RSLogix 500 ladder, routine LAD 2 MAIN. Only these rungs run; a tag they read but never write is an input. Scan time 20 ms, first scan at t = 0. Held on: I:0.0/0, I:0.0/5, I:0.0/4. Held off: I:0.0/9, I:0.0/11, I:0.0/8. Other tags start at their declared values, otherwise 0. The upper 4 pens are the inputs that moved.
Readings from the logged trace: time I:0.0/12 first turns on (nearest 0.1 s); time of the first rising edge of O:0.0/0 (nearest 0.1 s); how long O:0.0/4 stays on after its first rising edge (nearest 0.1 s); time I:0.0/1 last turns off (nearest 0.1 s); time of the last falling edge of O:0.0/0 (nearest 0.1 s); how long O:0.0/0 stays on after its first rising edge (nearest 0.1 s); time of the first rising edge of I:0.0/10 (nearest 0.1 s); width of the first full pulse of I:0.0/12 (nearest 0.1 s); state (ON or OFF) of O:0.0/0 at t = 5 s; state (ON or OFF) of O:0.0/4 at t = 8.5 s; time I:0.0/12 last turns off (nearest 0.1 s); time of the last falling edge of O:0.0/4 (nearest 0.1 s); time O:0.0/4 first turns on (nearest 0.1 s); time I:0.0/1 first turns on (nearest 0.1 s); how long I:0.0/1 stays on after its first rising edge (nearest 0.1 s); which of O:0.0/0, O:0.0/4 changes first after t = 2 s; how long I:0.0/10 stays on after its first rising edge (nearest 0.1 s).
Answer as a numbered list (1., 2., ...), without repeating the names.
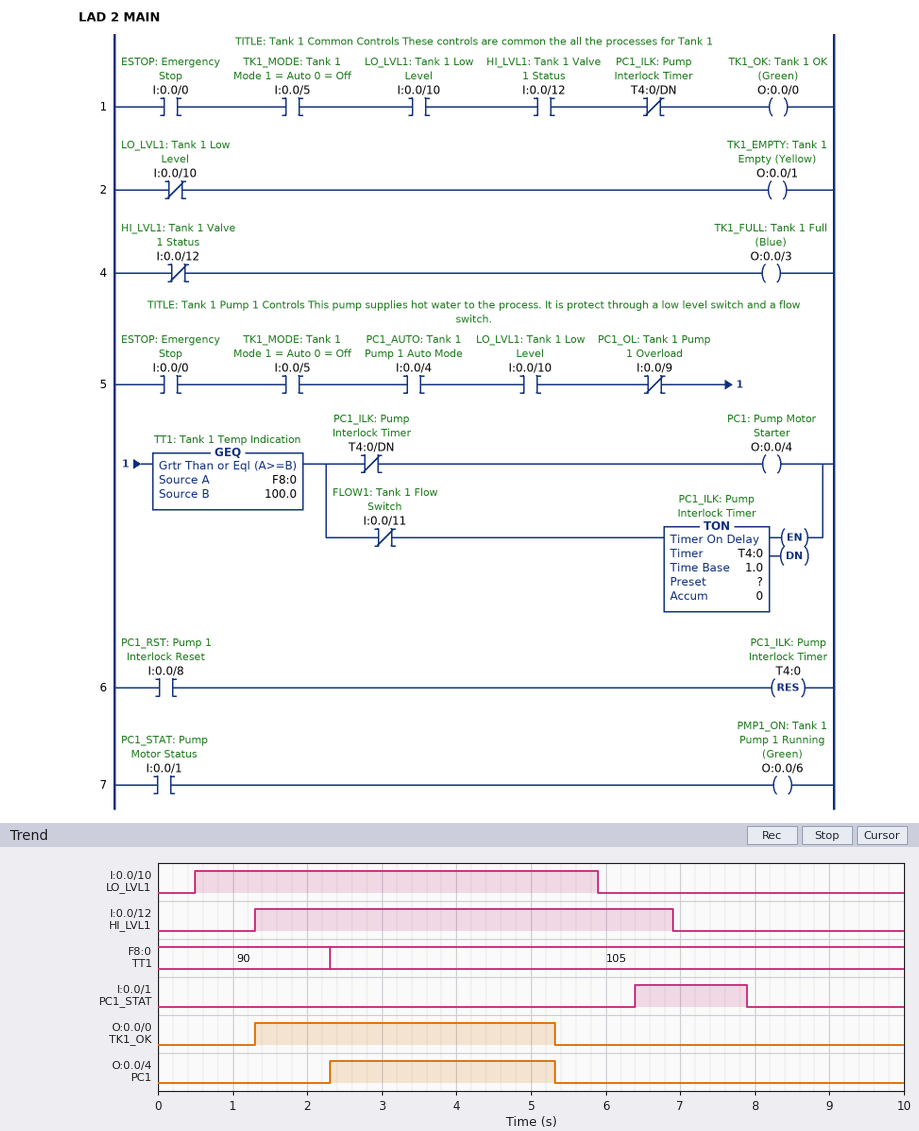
1. 1.3 s
2. 1.3 s
3. 3.0 s
4. 7.9 s
5. 5.3 s
6. 4.0 s
7. 0.5 s
8. 5.6 s
9. ON
10. OFF
11. 6.9 s
12. 5.3 s
13. 2.3 s
14. 6.4 s
15. 1.5 s
16. O:0.0/4
17. 5.4 s
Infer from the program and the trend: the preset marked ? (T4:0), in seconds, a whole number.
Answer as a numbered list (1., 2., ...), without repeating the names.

1. 3 s
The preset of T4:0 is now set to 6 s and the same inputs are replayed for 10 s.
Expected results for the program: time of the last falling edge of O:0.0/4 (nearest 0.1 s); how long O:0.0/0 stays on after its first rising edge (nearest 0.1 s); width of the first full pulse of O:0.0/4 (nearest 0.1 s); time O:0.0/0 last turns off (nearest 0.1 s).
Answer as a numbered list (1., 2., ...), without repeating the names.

1. 5.9 s
2. 4.6 s
3. 3.6 s
4. 5.9 s
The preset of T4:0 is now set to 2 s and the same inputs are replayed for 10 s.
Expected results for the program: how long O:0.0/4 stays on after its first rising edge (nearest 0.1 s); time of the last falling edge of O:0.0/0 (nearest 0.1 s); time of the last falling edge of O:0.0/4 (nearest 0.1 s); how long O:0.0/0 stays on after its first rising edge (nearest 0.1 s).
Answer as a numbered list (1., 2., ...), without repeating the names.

1. 2.0 s
2. 4.3 s
3. 4.3 s
4. 3.0 s
